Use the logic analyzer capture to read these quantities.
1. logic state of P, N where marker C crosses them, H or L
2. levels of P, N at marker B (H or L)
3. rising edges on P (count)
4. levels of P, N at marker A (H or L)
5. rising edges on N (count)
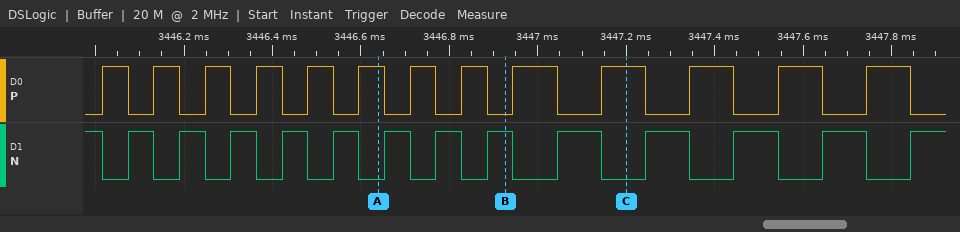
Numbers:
P=H, N=L
P=L, N=H
13
P=H, N=L
13
